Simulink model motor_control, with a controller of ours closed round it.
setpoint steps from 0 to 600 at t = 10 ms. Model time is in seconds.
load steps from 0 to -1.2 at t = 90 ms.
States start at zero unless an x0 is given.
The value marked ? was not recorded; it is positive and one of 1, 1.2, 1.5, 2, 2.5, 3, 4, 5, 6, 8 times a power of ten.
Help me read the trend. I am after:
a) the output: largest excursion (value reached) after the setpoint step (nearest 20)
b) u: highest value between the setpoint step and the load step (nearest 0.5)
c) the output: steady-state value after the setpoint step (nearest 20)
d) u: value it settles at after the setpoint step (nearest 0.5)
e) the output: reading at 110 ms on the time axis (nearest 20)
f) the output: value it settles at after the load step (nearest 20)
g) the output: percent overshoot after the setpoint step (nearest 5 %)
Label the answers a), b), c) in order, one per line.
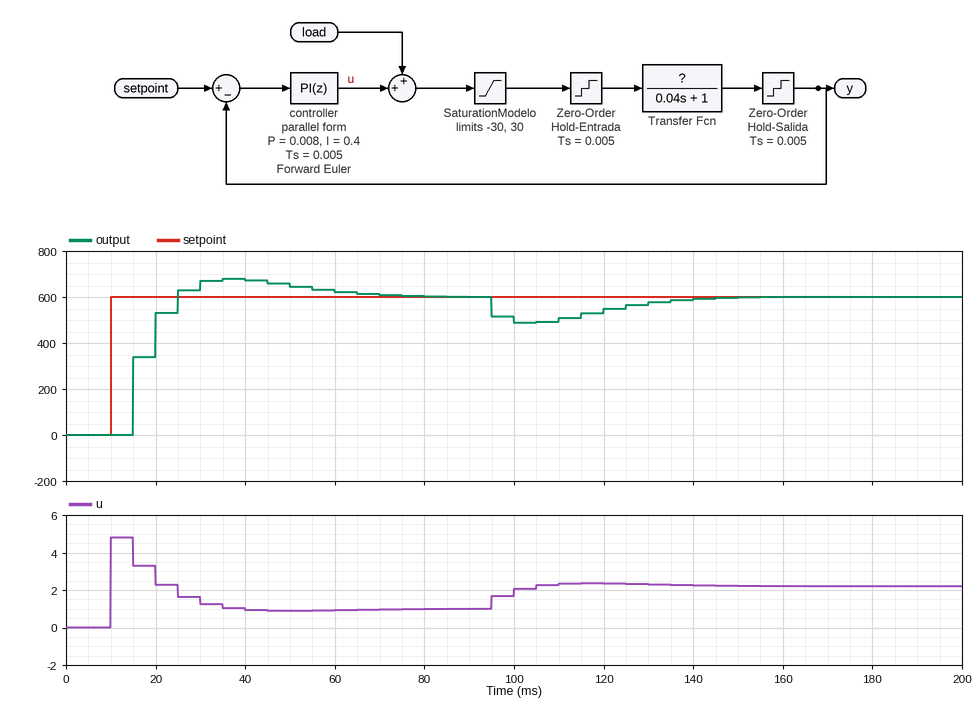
a) 680
b) 5.0
c) 600
d) 1.0
e) 500
f) 600
g) 15 %
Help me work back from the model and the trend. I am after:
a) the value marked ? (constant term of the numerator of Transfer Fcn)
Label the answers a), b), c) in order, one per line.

a) 600
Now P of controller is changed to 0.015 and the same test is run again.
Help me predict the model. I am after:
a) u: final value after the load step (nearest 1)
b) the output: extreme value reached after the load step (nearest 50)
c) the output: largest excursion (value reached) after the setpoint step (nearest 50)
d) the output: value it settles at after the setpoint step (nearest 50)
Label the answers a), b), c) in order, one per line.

a) 2
b) 500
c) 650
d) 600
